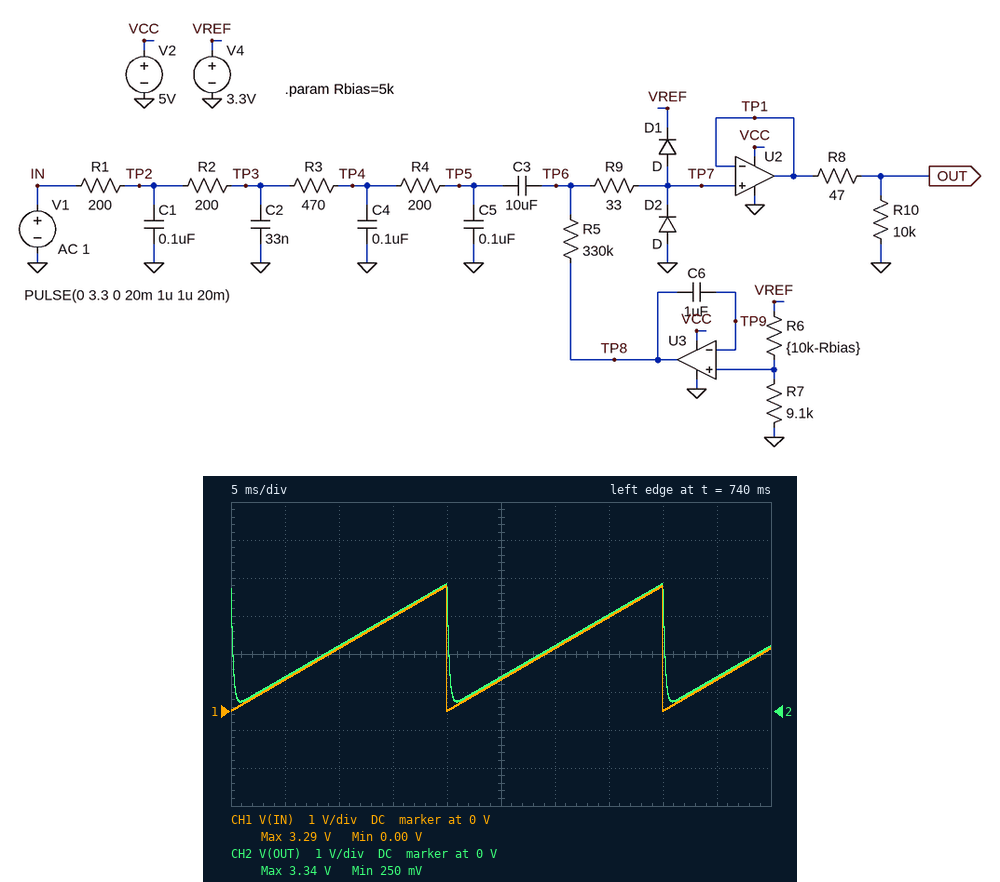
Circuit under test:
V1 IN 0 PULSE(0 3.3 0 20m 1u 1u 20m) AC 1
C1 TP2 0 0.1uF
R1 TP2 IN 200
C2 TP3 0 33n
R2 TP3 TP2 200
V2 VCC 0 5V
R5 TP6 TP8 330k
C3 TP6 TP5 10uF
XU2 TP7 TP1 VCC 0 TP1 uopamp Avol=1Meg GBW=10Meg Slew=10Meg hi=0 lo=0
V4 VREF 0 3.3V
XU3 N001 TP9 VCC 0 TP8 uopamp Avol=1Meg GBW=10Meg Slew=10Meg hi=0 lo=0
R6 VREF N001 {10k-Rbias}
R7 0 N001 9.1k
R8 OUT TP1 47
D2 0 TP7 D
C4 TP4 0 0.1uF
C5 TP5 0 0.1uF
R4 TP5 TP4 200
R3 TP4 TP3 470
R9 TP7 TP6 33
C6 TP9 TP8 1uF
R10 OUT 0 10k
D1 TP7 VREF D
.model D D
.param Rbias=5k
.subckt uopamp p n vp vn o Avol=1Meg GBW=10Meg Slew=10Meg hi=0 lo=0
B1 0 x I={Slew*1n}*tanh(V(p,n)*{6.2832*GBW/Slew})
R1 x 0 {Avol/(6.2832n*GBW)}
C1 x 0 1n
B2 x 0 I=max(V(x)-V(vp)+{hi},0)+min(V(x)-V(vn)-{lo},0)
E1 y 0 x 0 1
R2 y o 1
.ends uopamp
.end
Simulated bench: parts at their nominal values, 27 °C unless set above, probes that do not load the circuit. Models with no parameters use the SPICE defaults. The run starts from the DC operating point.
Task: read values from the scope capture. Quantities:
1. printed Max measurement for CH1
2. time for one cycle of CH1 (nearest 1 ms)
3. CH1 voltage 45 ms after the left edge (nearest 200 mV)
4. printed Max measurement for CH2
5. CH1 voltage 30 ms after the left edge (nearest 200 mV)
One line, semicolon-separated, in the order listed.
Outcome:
3.29 V; 20 ms; 800 mV; 3.34 V; 1.6 V
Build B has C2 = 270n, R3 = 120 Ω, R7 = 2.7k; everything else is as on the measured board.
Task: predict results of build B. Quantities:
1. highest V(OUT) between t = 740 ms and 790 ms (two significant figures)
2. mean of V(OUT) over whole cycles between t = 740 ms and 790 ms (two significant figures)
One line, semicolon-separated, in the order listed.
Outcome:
3.1 V; 1.5 V
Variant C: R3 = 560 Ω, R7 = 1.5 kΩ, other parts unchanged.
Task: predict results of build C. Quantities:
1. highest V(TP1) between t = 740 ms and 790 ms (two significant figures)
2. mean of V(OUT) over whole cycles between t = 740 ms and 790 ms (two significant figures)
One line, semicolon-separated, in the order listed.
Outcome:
3.1 V; 1.5 V
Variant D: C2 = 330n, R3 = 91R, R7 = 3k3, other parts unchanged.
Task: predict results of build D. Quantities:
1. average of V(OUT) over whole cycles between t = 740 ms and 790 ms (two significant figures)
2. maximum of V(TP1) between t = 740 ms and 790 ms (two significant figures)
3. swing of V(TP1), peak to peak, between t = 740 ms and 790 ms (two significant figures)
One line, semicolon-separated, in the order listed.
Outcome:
1.6 V; 3.2 V; 3.1 V
